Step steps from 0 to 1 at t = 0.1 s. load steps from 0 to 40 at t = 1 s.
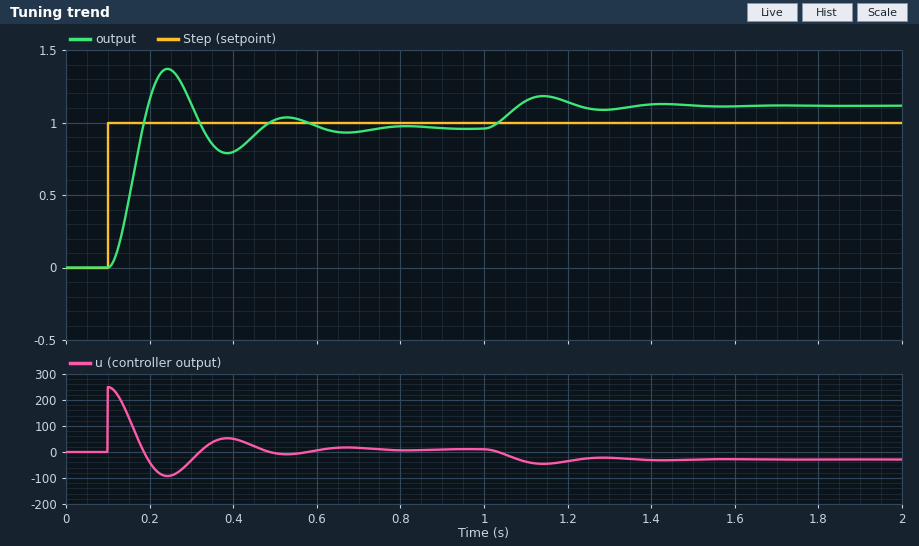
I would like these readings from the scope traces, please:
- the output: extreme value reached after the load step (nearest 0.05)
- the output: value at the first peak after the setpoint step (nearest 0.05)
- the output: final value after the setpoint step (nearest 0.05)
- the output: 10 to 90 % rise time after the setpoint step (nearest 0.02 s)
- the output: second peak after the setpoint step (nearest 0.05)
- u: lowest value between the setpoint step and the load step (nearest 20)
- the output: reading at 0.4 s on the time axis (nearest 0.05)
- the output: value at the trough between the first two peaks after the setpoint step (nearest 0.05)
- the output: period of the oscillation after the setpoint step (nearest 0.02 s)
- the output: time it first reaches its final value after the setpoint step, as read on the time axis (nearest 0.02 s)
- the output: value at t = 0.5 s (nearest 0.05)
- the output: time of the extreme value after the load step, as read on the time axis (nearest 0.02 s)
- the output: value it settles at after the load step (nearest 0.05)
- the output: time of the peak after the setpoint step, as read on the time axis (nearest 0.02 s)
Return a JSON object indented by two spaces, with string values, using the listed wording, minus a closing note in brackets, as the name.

{
  "the output: extreme value reached after the load step": "1.20",
  "the output: value at the first peak after the setpoint step": "1.35",
  "the output: final value after the setpoint step": "0.95",
  "the output: 10 to 90 % rise time after the setpoint step": "0.06 s",
  "the output: second peak after the setpoint step": "1.05",
  "u: lowest value between the setpoint step and the load step": "-100",
  "the output: reading at 0.4 s on the time axis": "0.80",
  "the output: value at the trough between the first two peaks after the setpoint step": "0.80",
  "the output: period of the oscillation after the setpoint step": "0.28 s",
  "the output: time it first reaches its final value after the setpoint step, as read on the time axis": "0.18 s",
  "the output: value at t = 0.5 s": "1.00",
  "the output: time of the extreme value after the load step, as read on the time axis": "1.14 s",
  "the output: value it settles at after the load step": "1.10",
  "the output: time of the peak after the setpoint step, as read on the time axis": "0.24 s"
}
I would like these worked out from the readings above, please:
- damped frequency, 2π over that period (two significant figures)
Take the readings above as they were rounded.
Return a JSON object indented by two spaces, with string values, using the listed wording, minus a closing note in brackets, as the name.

{
  "damped frequency, 2π over that period": "22 rad/s"
}
